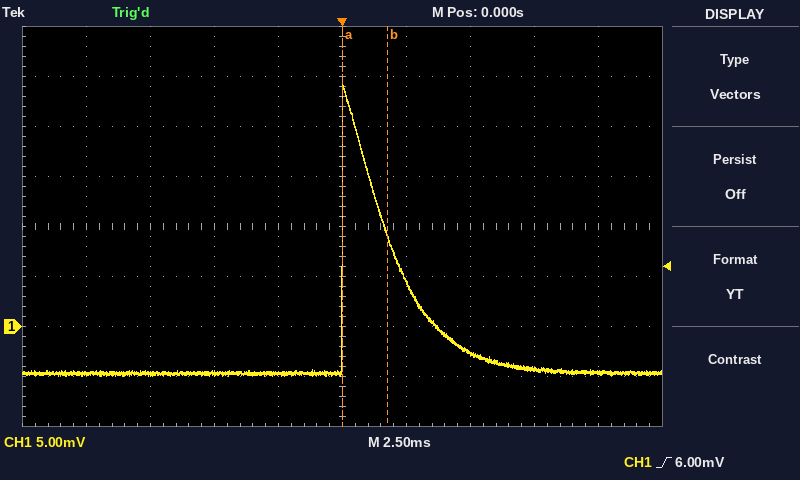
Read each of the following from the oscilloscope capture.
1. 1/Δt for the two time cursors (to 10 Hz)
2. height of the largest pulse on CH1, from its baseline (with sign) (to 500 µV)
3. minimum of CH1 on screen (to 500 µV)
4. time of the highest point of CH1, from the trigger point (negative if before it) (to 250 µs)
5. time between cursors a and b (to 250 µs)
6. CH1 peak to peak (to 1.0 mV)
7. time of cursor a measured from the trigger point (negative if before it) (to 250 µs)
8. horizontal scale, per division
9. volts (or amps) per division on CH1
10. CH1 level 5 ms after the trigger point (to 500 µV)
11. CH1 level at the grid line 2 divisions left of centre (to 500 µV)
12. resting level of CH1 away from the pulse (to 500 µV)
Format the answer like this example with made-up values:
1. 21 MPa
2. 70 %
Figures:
1. 570 Hz
2. +29.0 mV
3. -5.0 mV
4. 0.00 ms
5. 1.75 ms
6. 29.0 mV
7. 0.00 ms
8. 2.5 ms
9. 5 mV
10. -2.5 mV
11. -4.5 mV
12. -4.5 mV
